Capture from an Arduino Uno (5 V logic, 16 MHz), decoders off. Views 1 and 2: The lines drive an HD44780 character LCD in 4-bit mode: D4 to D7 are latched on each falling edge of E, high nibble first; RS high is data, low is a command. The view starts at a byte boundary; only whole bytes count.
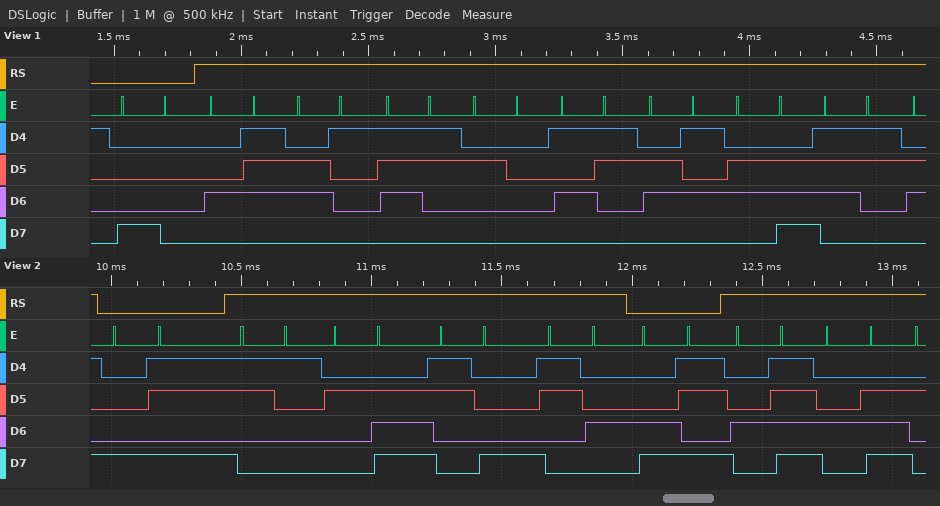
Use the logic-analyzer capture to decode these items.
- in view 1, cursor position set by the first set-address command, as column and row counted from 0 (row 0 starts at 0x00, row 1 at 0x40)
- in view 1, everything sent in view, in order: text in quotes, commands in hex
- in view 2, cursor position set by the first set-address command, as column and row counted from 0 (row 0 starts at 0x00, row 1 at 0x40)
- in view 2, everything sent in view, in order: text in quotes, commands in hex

column 0, row 0
0x80 "Gas Sens"
column 11, row 0
0x8B "1.84" 0xCB "ON"
